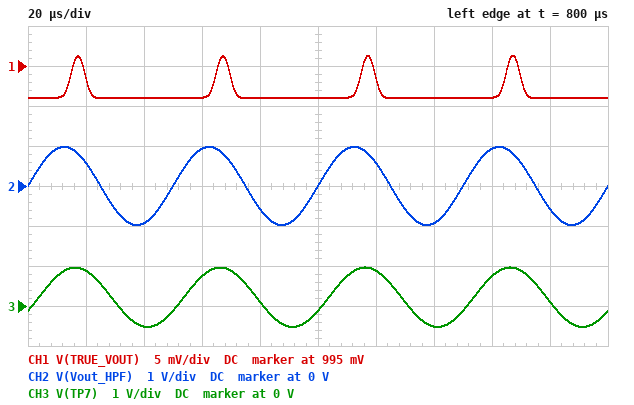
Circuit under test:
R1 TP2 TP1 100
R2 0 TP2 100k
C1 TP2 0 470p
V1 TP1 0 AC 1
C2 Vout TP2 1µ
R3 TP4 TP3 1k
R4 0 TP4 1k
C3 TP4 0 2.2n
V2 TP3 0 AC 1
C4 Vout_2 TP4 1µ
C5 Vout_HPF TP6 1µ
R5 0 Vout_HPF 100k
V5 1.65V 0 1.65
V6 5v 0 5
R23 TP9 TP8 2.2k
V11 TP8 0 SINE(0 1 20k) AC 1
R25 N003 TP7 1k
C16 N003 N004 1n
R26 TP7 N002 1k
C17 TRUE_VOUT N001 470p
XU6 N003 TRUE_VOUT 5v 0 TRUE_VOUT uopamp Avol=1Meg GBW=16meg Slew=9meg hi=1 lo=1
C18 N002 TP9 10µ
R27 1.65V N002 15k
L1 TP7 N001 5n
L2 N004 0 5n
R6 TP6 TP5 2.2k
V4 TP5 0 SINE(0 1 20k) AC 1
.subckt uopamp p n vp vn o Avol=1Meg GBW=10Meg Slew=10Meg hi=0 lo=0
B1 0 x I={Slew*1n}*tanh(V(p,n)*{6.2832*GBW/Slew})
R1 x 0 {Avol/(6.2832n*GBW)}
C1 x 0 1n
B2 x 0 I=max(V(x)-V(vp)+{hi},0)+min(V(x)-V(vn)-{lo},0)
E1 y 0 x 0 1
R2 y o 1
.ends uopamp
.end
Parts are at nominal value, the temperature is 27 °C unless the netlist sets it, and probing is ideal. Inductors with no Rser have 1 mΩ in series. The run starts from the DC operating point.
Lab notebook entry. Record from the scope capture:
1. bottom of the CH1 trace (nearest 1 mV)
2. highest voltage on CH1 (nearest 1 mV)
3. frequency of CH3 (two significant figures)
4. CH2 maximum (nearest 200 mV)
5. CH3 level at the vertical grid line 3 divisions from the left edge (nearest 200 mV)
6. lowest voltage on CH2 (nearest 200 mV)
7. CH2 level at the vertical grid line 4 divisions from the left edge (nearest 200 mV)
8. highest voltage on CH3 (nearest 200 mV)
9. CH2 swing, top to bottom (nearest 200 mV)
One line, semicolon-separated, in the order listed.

991 mV; 996 mV; 20 kHz; 1.0 V; 800 mV; -1.0 V; -600 mV; 1.0 V; 2.0 V
